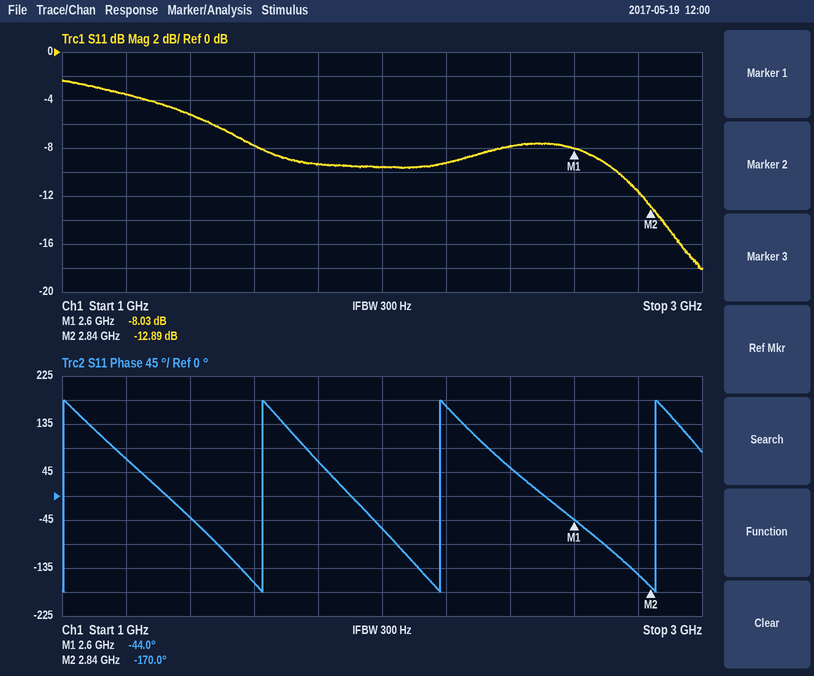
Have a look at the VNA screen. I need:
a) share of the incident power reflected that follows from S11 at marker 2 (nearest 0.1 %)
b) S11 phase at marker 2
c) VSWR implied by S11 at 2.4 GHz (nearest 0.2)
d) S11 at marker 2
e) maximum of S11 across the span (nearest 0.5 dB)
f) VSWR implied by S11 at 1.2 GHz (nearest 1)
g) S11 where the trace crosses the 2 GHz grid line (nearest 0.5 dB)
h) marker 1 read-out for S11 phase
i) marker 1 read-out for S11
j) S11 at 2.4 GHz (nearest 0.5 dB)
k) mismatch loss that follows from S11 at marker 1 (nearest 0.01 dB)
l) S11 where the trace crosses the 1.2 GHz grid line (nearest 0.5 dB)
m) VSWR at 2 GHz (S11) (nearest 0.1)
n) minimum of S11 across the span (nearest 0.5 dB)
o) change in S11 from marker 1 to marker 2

5.1 %
-170.0°
2.4
-12.89 dB
-2.5 dB
5
-9.5 dB
-44.0°
-8.03 dB
-8.0 dB
0.74 dB
-3.5 dB
2.0
-18.0 dB
-4.86 dB
